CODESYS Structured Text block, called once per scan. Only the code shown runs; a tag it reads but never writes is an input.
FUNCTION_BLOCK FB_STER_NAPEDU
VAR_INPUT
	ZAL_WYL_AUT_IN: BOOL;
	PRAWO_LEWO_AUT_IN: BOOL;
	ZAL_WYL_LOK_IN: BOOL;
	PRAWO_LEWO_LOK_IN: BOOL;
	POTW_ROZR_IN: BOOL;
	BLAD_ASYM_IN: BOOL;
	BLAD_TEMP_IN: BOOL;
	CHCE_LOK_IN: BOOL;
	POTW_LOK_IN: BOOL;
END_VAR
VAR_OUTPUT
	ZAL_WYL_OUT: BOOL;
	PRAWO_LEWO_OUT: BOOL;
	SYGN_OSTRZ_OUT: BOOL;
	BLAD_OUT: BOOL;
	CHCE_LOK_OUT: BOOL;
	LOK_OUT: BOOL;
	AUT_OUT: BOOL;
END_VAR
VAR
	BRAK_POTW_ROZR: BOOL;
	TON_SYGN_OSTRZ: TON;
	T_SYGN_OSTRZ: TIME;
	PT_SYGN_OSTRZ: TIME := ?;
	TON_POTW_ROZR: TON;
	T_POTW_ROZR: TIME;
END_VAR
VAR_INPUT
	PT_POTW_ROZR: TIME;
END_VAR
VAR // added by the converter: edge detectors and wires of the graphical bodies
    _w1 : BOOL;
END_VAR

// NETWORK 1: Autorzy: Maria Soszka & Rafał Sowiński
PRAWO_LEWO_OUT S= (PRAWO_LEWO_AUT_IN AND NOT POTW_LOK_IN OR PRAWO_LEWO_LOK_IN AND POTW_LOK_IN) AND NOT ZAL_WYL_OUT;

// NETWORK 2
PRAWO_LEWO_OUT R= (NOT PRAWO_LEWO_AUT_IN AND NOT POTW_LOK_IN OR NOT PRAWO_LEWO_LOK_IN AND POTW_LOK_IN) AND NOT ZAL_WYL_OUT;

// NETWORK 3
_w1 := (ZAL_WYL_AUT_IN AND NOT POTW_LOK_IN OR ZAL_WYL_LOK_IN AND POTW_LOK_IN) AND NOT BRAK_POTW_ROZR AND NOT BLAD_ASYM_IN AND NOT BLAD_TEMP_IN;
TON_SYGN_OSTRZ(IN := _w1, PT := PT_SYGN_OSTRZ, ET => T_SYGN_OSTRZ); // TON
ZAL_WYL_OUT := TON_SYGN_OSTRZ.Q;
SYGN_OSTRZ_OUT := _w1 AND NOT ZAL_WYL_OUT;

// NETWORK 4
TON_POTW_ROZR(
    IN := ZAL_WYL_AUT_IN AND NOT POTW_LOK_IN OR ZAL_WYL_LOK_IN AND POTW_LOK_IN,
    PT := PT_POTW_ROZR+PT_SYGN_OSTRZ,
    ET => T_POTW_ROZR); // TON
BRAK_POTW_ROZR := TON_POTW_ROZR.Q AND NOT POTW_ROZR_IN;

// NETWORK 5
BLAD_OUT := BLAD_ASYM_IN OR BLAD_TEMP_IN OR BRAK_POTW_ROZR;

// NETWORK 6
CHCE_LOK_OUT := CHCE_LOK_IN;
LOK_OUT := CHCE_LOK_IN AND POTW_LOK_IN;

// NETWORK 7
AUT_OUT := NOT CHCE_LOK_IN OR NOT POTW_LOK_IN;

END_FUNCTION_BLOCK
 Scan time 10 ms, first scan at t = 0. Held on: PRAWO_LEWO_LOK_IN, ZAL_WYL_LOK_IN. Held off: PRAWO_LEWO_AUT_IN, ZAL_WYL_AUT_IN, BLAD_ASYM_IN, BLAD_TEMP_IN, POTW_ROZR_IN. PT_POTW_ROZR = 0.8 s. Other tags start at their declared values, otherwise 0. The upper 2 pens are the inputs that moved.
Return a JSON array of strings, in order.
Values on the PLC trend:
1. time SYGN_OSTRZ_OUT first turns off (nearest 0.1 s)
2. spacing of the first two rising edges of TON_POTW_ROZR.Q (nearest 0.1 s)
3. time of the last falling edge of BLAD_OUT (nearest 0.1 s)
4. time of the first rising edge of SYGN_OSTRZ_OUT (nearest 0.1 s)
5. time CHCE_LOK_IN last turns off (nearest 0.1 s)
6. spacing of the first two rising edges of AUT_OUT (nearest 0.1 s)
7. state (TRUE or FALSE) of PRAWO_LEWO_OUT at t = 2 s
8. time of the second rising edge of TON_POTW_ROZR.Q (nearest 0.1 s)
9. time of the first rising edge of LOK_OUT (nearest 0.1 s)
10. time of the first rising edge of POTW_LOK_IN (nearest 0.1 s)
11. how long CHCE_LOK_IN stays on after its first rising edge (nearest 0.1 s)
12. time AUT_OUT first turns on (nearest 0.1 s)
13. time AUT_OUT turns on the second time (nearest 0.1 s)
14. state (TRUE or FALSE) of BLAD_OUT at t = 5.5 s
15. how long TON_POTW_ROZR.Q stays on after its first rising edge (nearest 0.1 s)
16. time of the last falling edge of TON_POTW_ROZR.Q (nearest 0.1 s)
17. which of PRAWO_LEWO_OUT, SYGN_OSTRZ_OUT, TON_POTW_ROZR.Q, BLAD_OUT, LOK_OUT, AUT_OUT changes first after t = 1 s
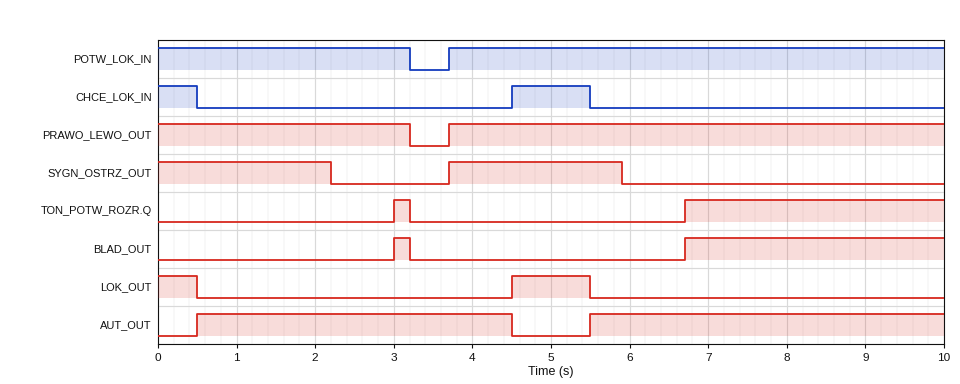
["2.2 s", "3.7 s", "3.2 s", "3.7 s", "5.5 s", "5.0 s", "TRUE", "6.7 s", "4.5 s", "3.7 s", "1.0 s", "0.5 s", "5.5 s", "FALSE", "0.2 s", "3.2 s", "SYGN_OSTRZ_OUT"]
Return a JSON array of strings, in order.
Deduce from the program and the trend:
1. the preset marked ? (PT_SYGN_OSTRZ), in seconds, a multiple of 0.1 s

["2.2 s"]
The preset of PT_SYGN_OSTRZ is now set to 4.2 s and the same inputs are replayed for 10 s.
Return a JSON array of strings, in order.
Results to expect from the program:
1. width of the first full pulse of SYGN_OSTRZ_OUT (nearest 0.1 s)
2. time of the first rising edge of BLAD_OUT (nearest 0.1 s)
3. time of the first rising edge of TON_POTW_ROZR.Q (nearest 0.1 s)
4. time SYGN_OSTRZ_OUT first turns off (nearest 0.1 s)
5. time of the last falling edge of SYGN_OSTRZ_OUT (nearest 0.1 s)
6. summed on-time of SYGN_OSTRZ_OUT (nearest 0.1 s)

["4.2 s", "8.7 s", "8.7 s", "3.2 s", "7.9 s", "7.4 s"]
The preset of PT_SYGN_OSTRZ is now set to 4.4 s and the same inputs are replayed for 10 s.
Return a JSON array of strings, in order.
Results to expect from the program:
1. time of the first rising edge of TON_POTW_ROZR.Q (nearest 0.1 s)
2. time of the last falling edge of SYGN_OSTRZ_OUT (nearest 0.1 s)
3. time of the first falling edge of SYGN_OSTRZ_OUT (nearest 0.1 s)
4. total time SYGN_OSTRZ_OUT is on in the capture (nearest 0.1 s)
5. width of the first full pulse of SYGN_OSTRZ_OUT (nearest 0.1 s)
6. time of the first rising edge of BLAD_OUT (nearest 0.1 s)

["8.9 s", "8.1 s", "3.2 s", "7.6 s", "4.4 s", "8.9 s"]
